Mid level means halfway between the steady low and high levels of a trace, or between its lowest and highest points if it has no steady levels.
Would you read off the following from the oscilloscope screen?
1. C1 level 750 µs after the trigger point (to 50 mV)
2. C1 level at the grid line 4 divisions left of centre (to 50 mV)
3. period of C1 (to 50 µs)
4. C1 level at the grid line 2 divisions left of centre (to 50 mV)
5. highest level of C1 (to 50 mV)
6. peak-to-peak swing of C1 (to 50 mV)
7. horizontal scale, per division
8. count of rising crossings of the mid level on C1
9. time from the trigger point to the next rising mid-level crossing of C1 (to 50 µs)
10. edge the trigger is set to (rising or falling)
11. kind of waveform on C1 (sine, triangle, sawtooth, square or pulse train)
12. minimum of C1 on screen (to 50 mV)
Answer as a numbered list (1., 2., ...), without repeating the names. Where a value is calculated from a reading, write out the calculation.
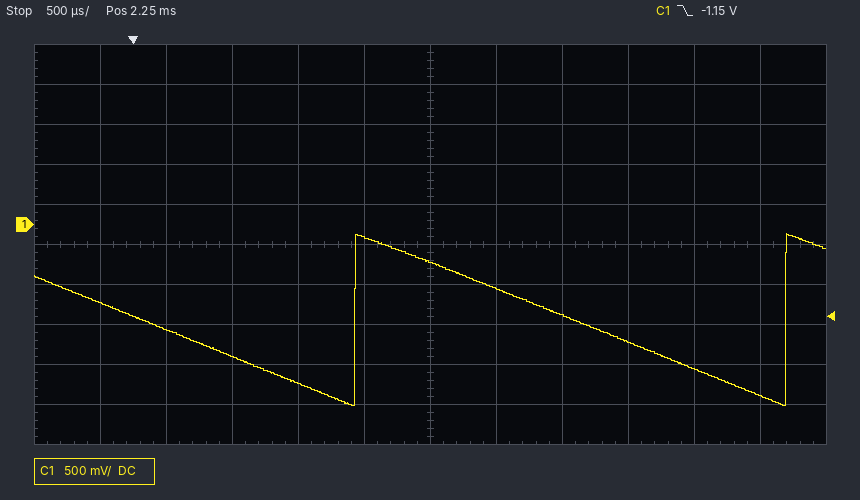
1. -1.65 V
2. -1.30 V
3. 3.25 ms
4. -2.00 V
5. -100 mV
6. -100 mV − (-2.25 V) = 2.15 V
7. 500 µs
8. 2
9. 1.70 ms
10. falling
11. sawtooth
12. -2.25 V
